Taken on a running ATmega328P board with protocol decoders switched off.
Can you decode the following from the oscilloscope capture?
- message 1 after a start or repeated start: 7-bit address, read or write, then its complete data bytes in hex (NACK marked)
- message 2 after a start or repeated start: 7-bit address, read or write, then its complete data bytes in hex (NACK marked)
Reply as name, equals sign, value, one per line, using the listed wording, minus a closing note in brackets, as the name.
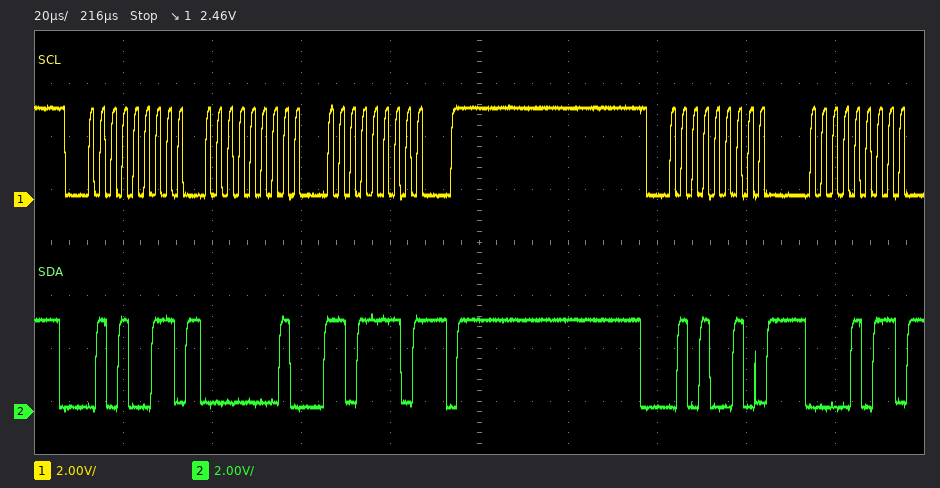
message 1 after a start or repeated start: 7-bit address, read or write, then its complete data bytes in hex = 0x29 read: 01 DE NACK
message 2 after a start or repeated start: 7-bit address, read or write, then its complete data bytes in hex = 0x29 write: 0B
